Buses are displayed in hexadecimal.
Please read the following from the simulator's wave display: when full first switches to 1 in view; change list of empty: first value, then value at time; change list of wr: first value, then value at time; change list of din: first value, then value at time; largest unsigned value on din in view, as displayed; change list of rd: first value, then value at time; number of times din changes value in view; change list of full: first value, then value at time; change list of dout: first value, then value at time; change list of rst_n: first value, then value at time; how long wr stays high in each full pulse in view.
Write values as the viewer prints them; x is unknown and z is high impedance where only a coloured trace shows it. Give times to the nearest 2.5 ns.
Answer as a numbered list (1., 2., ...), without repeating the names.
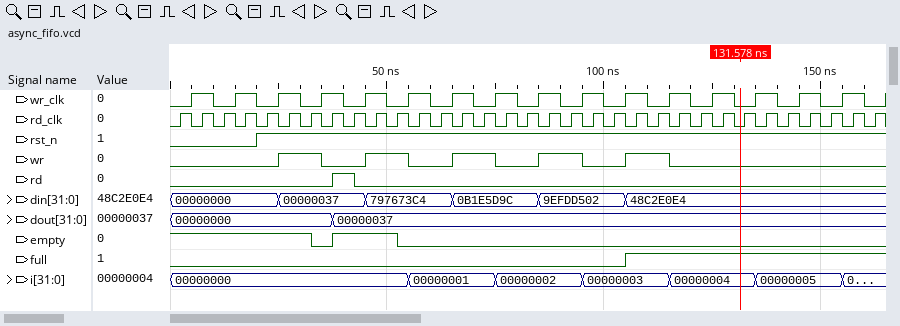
1. 105 ns
2. 1, 0 at 32.5 ns, 1 at 37.5 ns, 0 at 52.5 ns
3. 0, 1 at 25 ns, 0 at 35 ns, 1 at 45 ns, 0 at 55 ns, 1 at 65 ns, 0 at 75 ns, 1 at 85 ns, 0 at 95 ns, 1 at 105 ns, 0 at 115 ns
4. 00000000, 00000037 at 25 ns, 797673C4 at 45 ns, 0B1E5D9C at 65 ns, 9EFDD502 at 85 ns, 48C2E0E4 at 105 ns
5. 9EFDD502
6. 0, 1 at 37.5 ns, 0 at 42.5 ns
7. 5
8. 0, 1 at 105 ns
9. 00000000, 00000037 at 37.5 ns
10. 0, 1 at 20 ns
11. 10 ns, 10 ns, 10 ns, 10 ns, 10 ns
